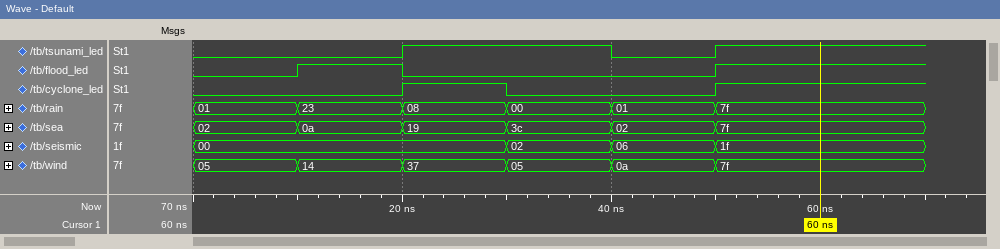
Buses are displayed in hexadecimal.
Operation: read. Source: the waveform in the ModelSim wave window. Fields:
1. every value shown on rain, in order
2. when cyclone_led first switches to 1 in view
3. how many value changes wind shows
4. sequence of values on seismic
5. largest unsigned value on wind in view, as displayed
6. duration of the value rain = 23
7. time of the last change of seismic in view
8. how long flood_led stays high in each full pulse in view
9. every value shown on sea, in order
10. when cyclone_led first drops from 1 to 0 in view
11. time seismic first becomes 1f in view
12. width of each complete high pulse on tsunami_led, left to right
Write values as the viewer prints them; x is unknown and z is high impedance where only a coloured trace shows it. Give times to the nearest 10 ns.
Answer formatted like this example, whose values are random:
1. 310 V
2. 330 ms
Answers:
1. 01, 23, 08, 00, 01, 7f
2. 20 ns
3. 5
4. 00, 02, 06, 1f
5. 7f
6. 10 ns
7. 50 ns
8. 10 ns
9. 02, 0a, 19, 3c, 02, 7f
10. 30 ns
11. 50 ns
12. 20 ns
